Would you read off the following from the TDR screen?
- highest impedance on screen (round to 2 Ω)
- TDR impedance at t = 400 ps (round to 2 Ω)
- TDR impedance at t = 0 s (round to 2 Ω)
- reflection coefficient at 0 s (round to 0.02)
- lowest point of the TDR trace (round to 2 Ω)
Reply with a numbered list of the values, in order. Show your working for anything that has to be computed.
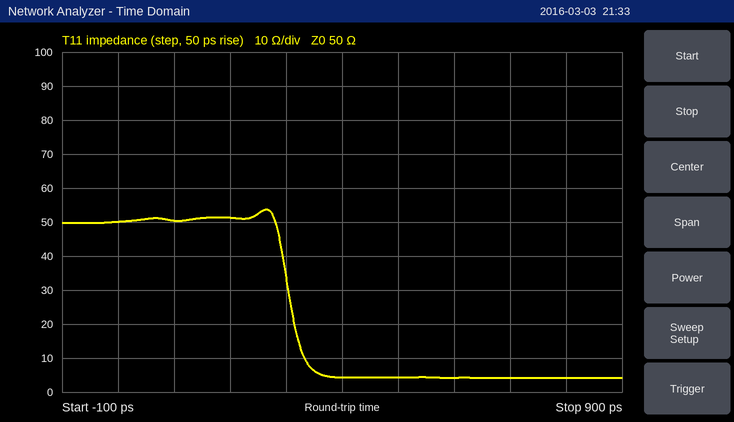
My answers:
1. 54 Ω
2. 4 Ω
3. 50 Ω
4. (50 − 50)/(50 + 50) ≈ 0.00
5. 4 Ω
